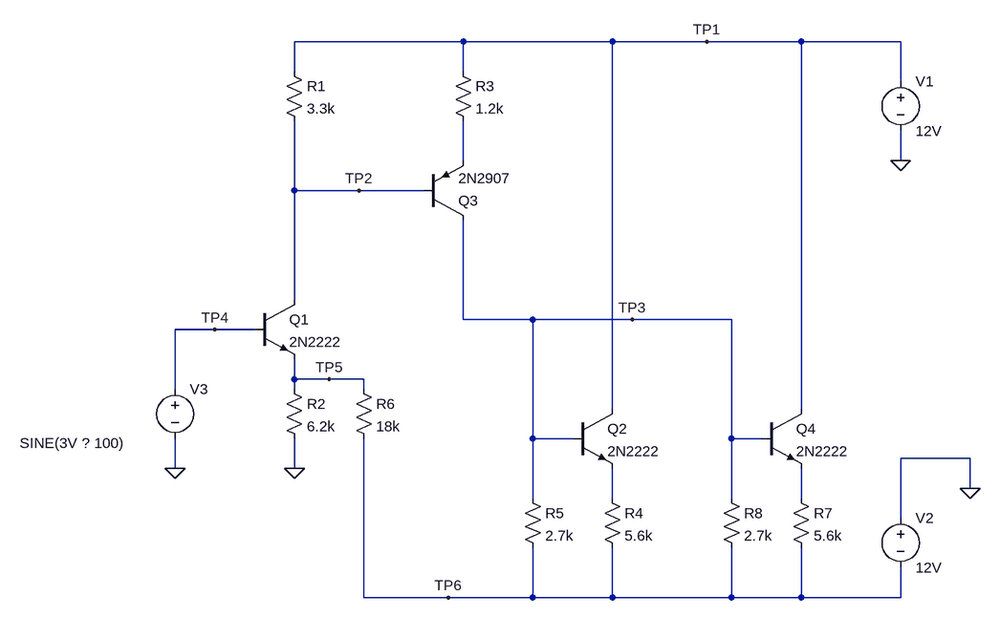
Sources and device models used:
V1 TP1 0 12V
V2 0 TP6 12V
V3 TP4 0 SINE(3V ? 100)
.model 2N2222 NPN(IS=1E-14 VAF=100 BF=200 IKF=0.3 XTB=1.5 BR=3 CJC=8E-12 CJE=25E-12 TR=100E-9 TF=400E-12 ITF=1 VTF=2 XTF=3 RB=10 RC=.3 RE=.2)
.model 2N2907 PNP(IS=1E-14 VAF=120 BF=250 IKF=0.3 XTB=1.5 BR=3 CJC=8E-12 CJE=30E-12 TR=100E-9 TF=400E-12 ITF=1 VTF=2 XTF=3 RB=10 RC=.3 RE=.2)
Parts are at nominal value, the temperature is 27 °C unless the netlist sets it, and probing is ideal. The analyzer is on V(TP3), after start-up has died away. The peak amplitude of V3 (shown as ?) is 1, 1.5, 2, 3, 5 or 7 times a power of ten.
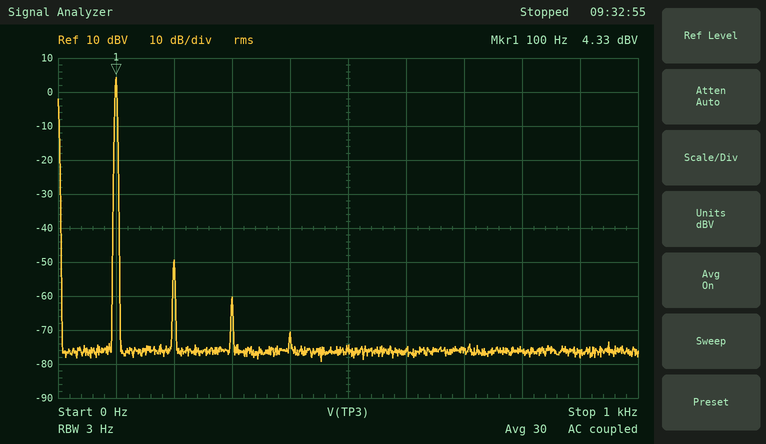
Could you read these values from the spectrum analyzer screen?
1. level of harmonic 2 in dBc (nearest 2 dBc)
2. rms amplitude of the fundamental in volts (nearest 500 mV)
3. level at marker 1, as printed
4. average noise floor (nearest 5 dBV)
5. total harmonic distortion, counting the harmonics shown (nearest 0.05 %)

-54 dBc
1.5 V
4.33 dBV
-75 dBV
0.20 %
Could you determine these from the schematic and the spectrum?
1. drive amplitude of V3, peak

3 V
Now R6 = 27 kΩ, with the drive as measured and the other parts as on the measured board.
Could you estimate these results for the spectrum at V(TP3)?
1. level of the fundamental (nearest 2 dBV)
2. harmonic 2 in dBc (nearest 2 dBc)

4 dBV
-48 dBc
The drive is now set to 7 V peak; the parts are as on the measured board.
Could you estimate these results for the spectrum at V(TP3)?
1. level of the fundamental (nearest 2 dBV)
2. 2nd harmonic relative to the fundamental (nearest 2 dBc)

4 dBV
-4 dBc
